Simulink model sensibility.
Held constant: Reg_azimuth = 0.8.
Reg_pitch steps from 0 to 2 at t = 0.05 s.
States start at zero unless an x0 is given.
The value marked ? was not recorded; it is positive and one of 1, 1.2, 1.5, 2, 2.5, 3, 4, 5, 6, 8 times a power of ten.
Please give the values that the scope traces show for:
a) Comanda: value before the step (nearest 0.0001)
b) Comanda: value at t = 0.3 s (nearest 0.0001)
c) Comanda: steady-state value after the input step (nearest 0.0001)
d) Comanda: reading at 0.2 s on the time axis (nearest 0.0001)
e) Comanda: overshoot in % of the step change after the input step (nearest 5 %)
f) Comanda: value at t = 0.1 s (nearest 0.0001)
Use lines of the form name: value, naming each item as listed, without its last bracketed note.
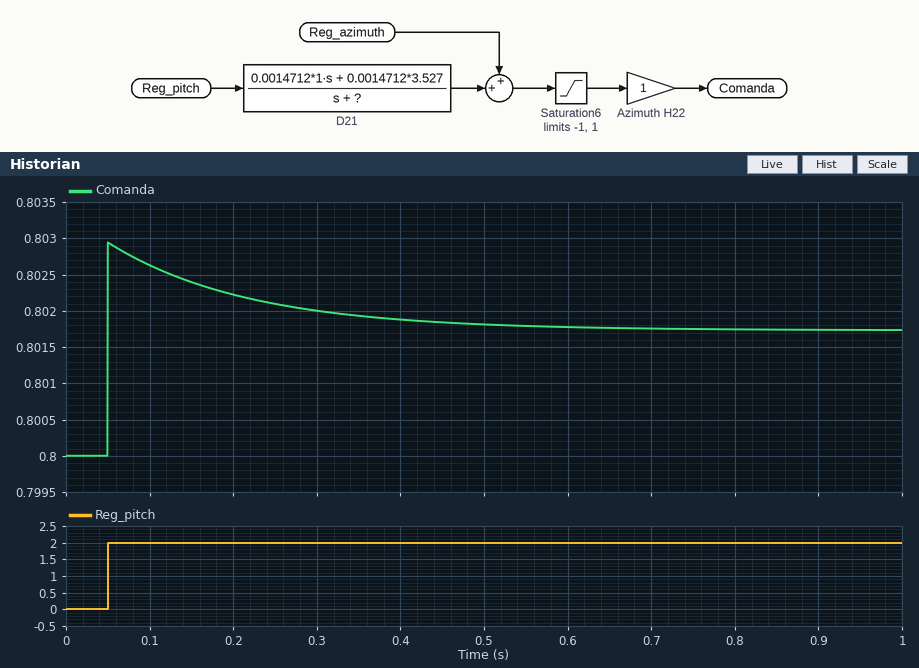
Comanda: value before the step: 0.8000
Comanda: value at t = 0.3 s: 0.8020
Comanda: steady-state value after the input step: 0.8017
Comanda: reading at 0.2 s on the time axis: 0.8022
Comanda: overshoot in % of the step change after the input step: 70 %
Comanda: value at t = 0.1 s: 0.8026
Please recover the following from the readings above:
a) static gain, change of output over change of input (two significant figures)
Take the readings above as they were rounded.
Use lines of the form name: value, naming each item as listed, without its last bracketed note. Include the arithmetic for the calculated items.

static gain, change of output over change of input: (0.8017 - 0.8) / (2 - 0) = 0.00085
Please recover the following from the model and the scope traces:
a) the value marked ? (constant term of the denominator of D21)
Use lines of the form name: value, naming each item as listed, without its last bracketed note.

the value marked ?: 6
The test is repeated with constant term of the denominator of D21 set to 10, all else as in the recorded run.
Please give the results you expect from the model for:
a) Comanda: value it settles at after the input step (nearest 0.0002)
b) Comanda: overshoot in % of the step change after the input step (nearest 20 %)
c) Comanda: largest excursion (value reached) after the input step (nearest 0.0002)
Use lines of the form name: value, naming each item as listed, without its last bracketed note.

Comanda: value it settles at after the input step: 0.8010
Comanda: overshoot in % of the step change after the input step: 180 %
Comanda: largest excursion (value reached) after the input step: 0.8030
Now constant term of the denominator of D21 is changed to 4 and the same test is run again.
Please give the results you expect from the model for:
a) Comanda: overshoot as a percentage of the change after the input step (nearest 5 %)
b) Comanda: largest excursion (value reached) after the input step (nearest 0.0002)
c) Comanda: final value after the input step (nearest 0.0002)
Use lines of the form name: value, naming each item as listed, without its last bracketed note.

Comanda: overshoot as a percentage of the change after the input step: 15 %
Comanda: largest excursion (value reached) after the input step: 0.8030
Comanda: final value after the input step: 0.8026
